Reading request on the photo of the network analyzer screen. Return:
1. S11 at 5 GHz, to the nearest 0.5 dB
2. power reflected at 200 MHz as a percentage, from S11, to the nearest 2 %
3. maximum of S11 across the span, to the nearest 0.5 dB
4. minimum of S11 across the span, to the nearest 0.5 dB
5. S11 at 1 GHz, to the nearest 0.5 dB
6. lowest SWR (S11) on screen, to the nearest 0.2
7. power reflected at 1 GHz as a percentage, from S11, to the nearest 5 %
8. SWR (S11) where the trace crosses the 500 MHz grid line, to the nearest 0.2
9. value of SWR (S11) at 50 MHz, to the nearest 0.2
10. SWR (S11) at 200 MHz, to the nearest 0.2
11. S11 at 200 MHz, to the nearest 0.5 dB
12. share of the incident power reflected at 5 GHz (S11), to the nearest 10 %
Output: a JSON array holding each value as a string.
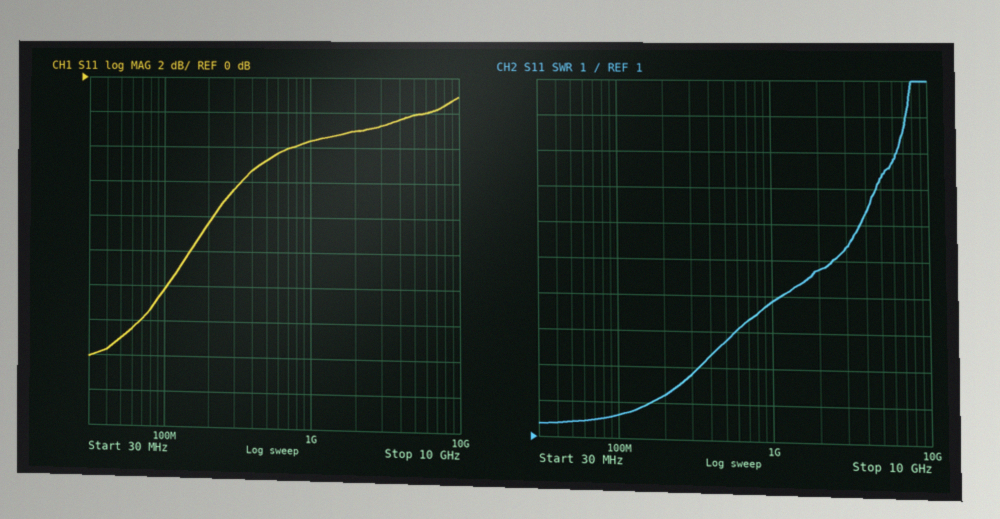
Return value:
["-2.0 dB", "14 %", "-1.0 dB", "-16.0 dB", "-3.5 dB", "1.4", "45 %", "3.8", "1.4", "2.2", "-8.5 dB", "60 %"]
